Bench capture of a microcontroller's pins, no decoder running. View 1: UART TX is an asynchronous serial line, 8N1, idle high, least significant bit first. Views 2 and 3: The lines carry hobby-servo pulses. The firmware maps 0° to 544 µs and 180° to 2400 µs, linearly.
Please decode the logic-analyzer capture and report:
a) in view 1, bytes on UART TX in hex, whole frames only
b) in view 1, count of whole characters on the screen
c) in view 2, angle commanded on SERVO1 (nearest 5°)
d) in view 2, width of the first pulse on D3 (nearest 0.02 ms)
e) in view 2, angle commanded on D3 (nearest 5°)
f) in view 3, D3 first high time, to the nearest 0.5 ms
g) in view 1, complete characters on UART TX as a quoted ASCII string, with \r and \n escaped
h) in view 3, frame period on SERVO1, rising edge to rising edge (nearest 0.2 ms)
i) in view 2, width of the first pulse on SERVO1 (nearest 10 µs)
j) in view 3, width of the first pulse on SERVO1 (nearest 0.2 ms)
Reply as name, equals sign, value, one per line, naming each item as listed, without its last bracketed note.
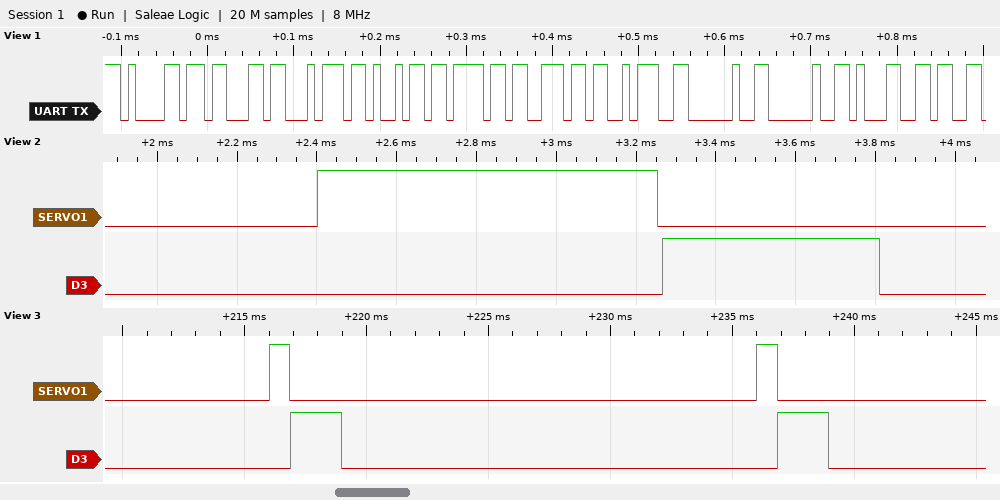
in view 1, bytes on UART TX in hex, whole frames only = 61 63 74 69 6F 6E 3A 20 20 31
in view 1, count of whole characters on the screen = 10
in view 2, angle commanded on SERVO1 = 30°
in view 2, width of the first pulse on D3 = 0.54 ms
in view 2, angle commanded on D3 = 0°
in view 3, D3 first high time, to the nearest 0.5 ms = 2.0 ms
in view 1, complete characters on UART TX as a quoted ASCII string, with \r and \n escaped = "action:  1"
in view 3, frame period on SERVO1, rising edge to rising edge = 20.0 ms
in view 2, width of the first pulse on SERVO1 = 850 µs
in view 3, width of the first pulse on SERVO1 = 0.8 ms
